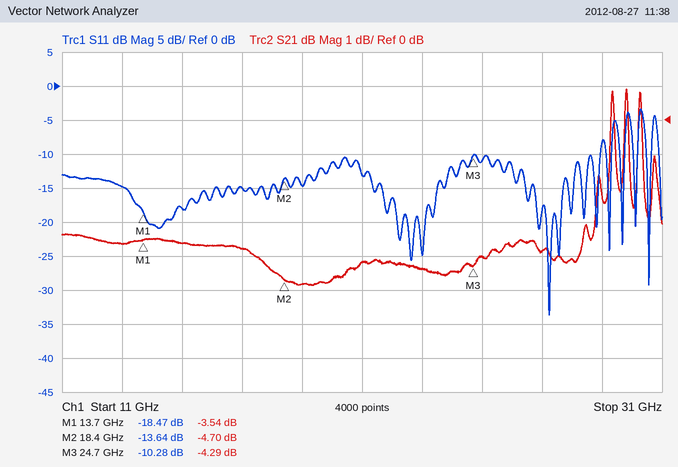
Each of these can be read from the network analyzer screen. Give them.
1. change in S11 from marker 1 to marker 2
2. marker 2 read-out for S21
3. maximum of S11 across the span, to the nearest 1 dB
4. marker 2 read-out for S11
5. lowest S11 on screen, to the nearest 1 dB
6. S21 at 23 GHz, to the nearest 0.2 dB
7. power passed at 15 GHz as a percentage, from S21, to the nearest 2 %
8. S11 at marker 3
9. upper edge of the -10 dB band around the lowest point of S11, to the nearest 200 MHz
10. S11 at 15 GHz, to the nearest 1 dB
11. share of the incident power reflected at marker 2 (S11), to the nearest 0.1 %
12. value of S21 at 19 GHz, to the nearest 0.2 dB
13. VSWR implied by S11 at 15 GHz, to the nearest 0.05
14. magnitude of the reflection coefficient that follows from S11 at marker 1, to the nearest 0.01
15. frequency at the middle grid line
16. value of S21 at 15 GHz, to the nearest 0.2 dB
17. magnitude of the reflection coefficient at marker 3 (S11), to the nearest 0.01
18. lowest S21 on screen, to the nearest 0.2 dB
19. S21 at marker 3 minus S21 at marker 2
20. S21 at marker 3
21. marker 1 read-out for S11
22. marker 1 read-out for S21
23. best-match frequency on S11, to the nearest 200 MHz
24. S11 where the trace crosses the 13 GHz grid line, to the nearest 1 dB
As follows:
4.83 dB
-4.70 dB
-3 dB
-13.64 dB
-34 dB
-4.4 dB
44 %
-10.28 dB
29.0 GHz
-18 dB
4.3 %
-4.8 dB
1.30
0.12
21 GHz
-3.6 dB
0.31
-4.8 dB
0.41 dB
-4.29 dB
-18.47 dB
-3.54 dB
27.2 GHz
-15 dB
